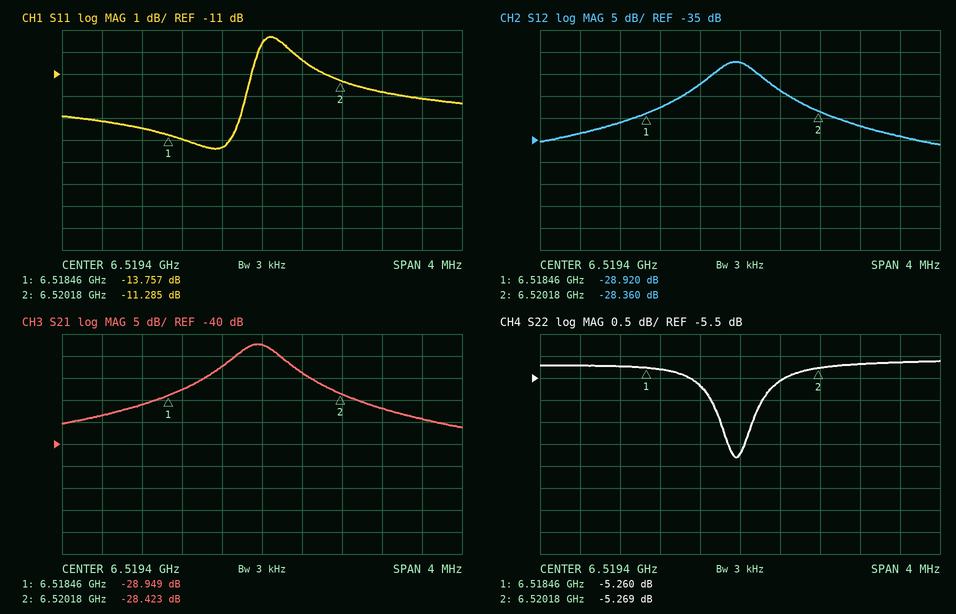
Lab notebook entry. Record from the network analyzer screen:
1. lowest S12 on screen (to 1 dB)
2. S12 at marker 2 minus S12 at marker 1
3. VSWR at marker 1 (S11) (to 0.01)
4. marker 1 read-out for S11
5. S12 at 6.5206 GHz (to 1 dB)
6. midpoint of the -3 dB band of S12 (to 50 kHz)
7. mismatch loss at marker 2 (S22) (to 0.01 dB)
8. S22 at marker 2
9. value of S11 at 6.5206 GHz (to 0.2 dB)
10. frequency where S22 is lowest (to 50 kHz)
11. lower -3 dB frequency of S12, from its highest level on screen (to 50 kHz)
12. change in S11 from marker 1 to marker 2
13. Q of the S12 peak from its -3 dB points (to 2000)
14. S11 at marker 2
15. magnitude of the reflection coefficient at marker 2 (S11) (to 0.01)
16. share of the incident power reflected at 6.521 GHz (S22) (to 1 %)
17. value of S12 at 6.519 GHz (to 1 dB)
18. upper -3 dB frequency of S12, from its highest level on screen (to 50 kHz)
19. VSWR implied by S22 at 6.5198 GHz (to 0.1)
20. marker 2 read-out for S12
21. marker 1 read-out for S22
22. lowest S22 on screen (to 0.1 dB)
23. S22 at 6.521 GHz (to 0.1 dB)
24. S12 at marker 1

-36 dB
0.560 dB
1.52
-13.757 dB
-32 dB
6.51935 GHz
1.53 dB
-5.269 dB
-11.8 dB
6.51935 GHz
6.51910 GHz
2.472 dB
14000
-11.285 dB
0.27
31 %
-22 dB
6.51960 GHz
3.2
-28.360 dB
-5.260 dB
-7.3 dB
-5.1 dB
-28.920 dB
